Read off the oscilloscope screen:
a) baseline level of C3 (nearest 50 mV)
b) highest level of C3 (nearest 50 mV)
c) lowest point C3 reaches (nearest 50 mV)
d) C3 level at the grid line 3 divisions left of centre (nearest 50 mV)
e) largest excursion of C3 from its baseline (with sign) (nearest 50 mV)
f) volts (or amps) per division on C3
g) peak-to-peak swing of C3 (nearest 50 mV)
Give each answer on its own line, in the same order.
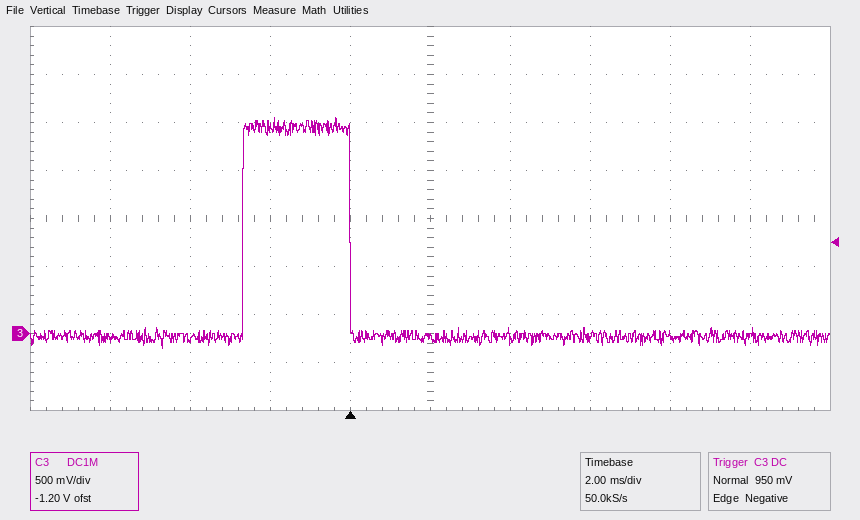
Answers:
-50 mV
2.25 V
-150 mV
-50 mV
+2.30 V
500 mV
2.40 V
